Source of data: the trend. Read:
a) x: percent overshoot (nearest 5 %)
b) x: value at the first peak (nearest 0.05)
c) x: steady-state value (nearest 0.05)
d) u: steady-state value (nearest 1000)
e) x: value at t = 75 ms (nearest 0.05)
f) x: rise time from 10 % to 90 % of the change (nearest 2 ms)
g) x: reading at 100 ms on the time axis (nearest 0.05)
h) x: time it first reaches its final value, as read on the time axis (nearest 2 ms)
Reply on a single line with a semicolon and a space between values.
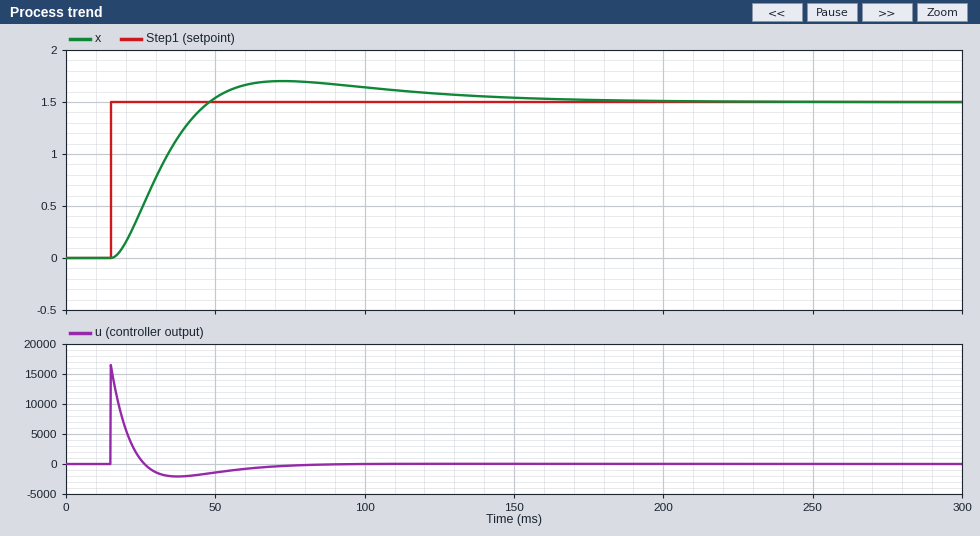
15 %; 1.70; 1.50; 0; 1.70; 22 ms; 1.65; 48 ms
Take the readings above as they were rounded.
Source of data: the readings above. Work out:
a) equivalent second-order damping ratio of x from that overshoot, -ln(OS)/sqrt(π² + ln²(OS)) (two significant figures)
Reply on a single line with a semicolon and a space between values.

0.52
